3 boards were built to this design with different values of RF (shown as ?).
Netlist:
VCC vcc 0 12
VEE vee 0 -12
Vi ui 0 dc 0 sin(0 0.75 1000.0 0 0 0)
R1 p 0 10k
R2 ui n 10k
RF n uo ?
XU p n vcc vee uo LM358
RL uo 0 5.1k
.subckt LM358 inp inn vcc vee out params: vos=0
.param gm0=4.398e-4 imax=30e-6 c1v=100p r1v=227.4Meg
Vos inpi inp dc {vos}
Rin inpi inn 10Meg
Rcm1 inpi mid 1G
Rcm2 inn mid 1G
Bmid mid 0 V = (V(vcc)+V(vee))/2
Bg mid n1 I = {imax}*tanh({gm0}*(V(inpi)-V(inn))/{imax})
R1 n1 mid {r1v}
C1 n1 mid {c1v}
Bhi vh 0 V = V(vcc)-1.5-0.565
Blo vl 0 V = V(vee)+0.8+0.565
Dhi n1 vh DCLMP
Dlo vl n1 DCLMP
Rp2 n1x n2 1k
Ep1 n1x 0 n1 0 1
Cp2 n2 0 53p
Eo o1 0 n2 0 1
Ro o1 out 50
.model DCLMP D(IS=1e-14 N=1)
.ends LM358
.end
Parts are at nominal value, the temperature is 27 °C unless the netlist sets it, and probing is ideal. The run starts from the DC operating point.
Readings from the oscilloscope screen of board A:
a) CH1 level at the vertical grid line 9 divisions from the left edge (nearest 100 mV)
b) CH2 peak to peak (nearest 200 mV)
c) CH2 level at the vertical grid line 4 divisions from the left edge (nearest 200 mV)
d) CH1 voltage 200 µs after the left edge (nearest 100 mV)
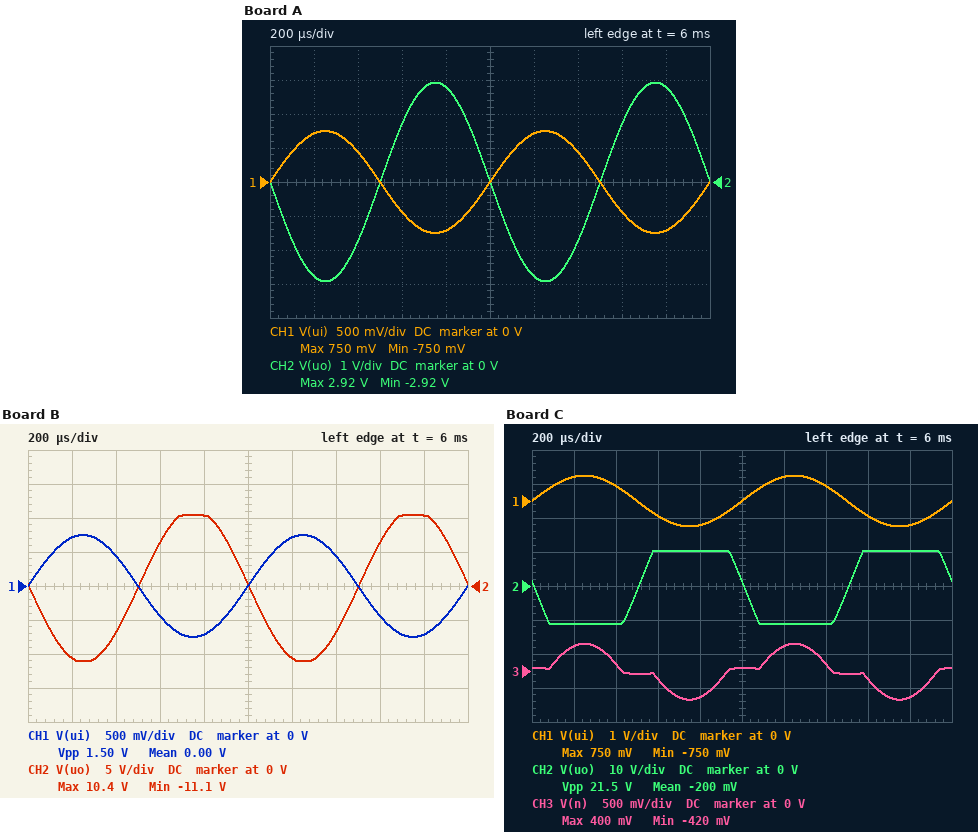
-700 mV
5.8 V
2.8 V
700 mV
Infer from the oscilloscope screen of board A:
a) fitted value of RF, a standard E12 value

39 kΩ
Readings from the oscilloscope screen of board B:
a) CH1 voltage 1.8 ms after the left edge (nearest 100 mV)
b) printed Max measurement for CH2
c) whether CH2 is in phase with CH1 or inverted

-700 mV
10.4 V
inverted
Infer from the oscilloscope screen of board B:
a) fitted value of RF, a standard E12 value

150 kΩ
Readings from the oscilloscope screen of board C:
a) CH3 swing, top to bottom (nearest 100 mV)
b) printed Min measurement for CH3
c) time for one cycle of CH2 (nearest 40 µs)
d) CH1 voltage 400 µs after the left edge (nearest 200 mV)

800 mV
-420 mV
1.00 ms
400 mV
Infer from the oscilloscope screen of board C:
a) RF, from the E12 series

330 kΩ
